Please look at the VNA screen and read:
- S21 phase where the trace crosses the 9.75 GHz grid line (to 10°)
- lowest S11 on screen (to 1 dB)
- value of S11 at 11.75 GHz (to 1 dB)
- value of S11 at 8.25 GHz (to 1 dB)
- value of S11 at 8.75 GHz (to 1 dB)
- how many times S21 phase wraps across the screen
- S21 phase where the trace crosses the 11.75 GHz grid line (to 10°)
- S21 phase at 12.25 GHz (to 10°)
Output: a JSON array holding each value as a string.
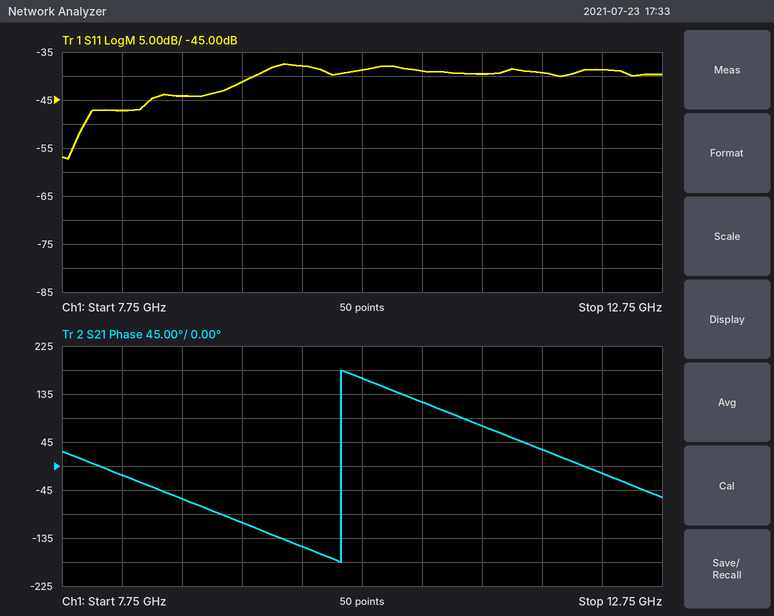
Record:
["-150°", "-57 dB", "-39 dB", "-47 dB", "-44 dB", "1", "30°", "-10°"]
